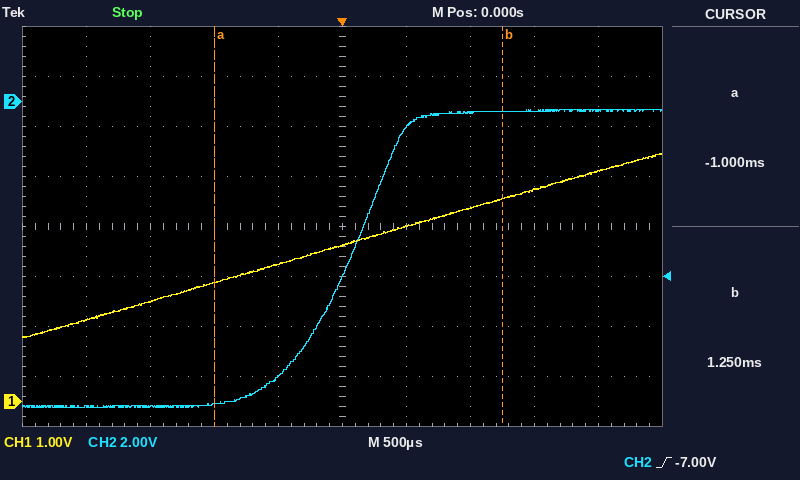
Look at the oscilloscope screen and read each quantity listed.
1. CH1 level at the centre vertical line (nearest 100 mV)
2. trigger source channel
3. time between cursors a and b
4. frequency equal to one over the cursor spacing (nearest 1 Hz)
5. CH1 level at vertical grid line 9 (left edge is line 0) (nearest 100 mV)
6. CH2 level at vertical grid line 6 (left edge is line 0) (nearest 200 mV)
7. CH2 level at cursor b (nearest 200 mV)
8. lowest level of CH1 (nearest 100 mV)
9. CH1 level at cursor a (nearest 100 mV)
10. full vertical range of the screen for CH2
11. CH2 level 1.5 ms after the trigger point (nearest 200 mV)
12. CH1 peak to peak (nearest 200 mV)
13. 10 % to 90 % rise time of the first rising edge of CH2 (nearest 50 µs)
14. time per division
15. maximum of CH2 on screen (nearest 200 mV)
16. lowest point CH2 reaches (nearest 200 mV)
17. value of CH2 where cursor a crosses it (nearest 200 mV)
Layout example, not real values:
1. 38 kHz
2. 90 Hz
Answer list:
1. 3.1 V
2. CH2
3. 2.25 ms
4. 444 Hz
5. 4.6 V
6. -1.0 V
7. -400 mV
8. 1.3 V
9. 2.4 V
10. 16 V
11. -400 mV
12. 3.6 V
13. 950 µs
14. 500 µs
15. -400 mV
16. -12.2 V
17. -12.2 V
